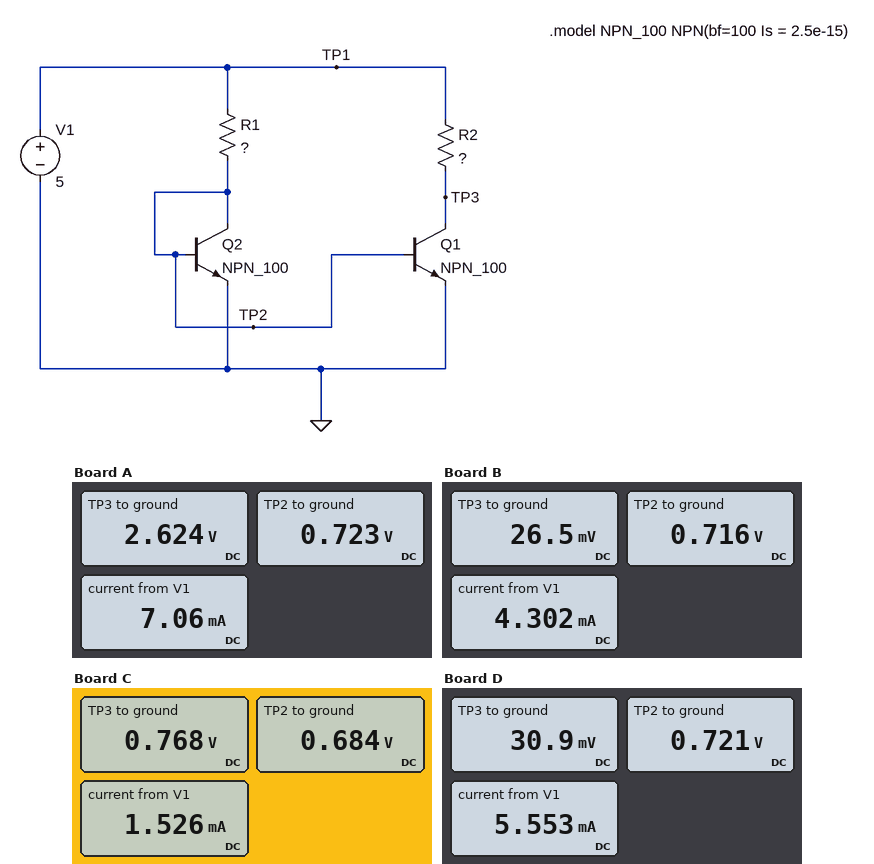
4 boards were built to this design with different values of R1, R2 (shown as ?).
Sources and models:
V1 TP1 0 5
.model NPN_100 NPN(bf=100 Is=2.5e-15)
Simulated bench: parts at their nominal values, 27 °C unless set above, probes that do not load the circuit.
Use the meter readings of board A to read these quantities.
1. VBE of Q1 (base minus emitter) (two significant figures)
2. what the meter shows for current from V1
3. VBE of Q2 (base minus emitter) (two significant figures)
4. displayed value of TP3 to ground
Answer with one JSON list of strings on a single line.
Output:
["720 mV", "7.06 mA", "720 mV", "2.624 V"]
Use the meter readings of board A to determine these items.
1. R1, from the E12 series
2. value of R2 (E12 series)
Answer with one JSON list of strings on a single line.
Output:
["1.2 kΩ", "680 Ω"]
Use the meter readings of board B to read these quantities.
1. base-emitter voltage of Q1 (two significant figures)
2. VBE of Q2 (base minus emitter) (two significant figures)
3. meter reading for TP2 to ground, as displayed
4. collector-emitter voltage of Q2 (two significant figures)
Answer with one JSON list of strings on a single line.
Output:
["720 mV", "720 mV", "0.716 V", "720 mV"]
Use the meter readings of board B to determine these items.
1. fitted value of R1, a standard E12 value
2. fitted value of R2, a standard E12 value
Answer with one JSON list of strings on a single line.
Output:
["1.2 kΩ", "6.8 kΩ"]
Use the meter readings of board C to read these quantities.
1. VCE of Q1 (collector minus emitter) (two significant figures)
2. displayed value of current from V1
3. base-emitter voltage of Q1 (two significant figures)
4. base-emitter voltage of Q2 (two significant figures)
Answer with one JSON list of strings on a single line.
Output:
["770 mV", "1.526 mA", "680 mV", "680 mV"]
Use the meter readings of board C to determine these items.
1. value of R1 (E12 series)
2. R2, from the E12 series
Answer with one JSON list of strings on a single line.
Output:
["5.6 kΩ", "5.6 kΩ"]
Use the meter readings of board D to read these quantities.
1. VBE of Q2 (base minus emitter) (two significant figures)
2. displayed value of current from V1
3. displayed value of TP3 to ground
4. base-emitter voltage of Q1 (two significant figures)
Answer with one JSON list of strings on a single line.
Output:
["720 mV", "5.553 mA", "30.9 mV", "720 mV"]
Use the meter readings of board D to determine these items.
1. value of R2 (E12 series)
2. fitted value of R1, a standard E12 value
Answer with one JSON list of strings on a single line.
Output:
["3.9 kΩ", "1 kΩ"]
